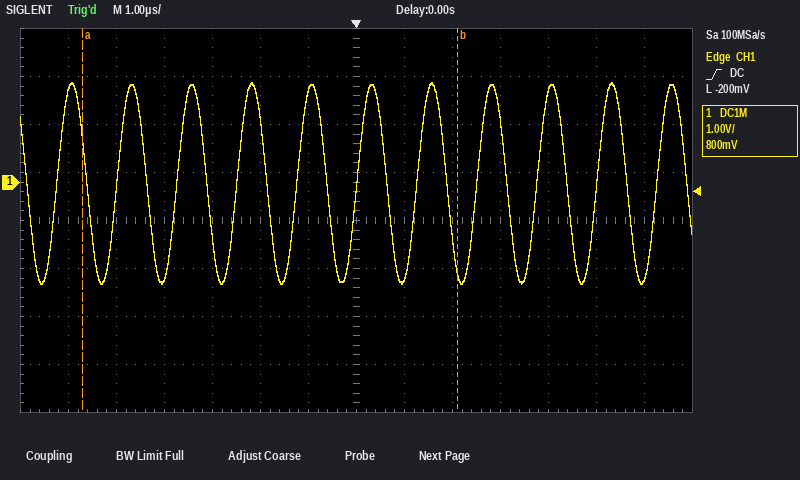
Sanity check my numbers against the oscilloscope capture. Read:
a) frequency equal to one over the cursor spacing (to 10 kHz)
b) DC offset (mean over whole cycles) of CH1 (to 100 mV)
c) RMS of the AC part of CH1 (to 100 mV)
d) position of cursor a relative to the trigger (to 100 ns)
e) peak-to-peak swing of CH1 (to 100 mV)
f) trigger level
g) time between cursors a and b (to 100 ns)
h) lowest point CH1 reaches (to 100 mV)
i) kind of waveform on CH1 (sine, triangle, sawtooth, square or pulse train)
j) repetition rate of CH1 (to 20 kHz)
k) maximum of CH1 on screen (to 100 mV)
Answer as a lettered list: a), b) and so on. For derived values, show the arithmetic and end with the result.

a) 1 / 7.8 µs ≈ 130 kHz
b) (2.1 V + (-2.1 V)) / 2 ≈ 0.0 V
c) 4.2 V / (2√2) ≈ 1.5 V
d) -5.7 µs
e) 2.1 V − (-2.1 V) = 4.2 V
f) -200 mV
g) 7.8 µs
h) -2.1 V
i) sine
j) 800 kHz
k) 2.1 V
